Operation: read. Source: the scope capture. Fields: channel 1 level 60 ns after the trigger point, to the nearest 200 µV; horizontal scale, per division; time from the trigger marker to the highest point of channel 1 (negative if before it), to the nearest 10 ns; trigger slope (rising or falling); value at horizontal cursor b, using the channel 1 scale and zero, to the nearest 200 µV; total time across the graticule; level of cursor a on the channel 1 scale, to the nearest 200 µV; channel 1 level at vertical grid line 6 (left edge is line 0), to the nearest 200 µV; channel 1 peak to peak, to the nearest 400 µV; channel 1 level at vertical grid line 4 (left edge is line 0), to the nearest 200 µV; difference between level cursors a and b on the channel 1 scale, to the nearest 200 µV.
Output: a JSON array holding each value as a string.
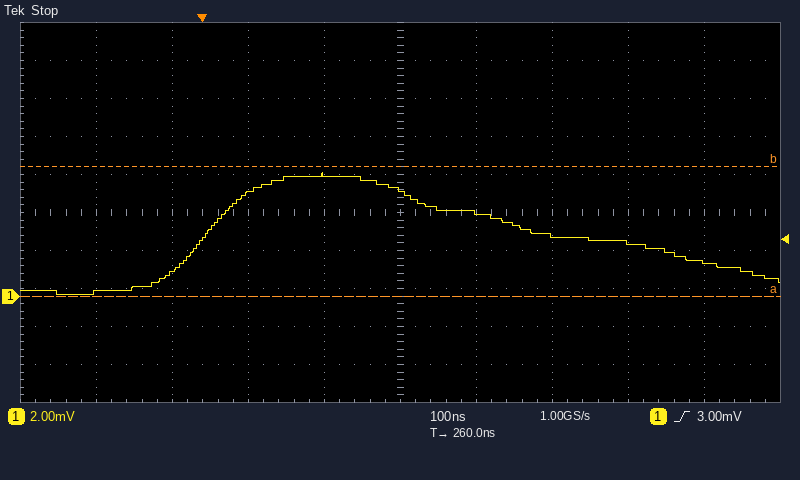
["5.4 mV", "100 ns", "+160 ns", "rising", "6.8 mV", "1 µs", "0.0 mV", "4.4 mV", "6.4 mV", "6.4 mV", "6.8 mV"]
